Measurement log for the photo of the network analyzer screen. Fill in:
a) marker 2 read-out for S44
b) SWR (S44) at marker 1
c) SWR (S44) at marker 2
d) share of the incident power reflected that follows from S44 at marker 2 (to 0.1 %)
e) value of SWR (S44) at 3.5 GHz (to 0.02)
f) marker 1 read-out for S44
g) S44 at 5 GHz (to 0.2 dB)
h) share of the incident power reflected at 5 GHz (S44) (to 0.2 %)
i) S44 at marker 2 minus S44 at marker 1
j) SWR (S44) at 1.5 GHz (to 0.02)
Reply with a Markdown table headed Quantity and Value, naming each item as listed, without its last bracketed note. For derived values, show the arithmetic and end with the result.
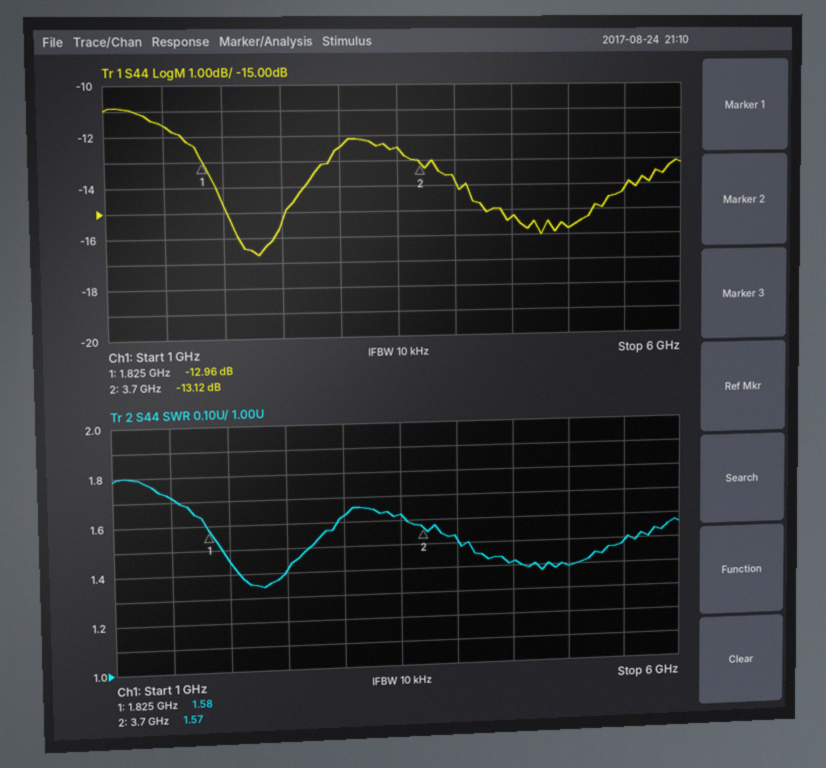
| Quantity | Value |
|---|---|
| marker 2 read-out for S44 | -13.12 dB |
| SWR (S44) at marker 1 | 1.58 |
| SWR (S44) at marker 2 | 1.57 |
| share of the incident power reflected that follows from S44 at marker 2 | 10^(-13.12/10) ≈ 4.9 % |
| value of SWR (S44) at 3.5 GHz | 1.62 |
| marker 1 read-out for S44 | -12.96 dB |
| S44 at 5 GHz | -15.8 dB |
| share of the incident power reflected at 5 GHz (S44) | 10^(-15.8/10) ≈ 2.6 % |
| S44 at marker 2 minus S44 at marker 1 | -13.12 − (-12.96) = -0.16 dB |
| SWR (S44) at 1.5 GHz | 1.72 |
